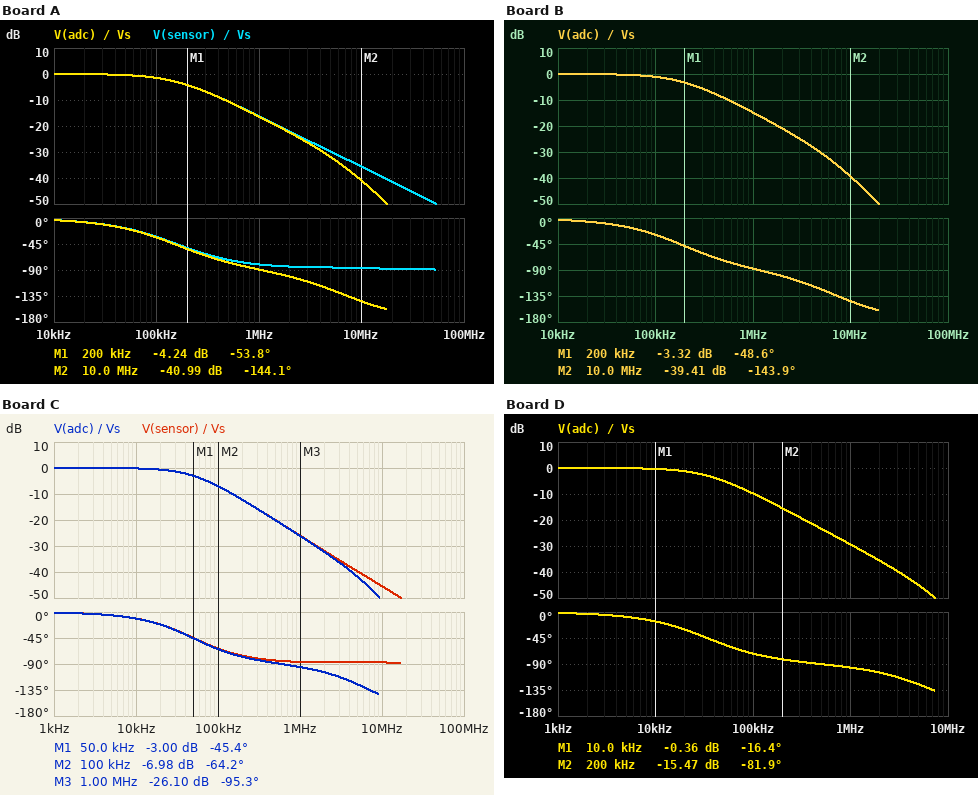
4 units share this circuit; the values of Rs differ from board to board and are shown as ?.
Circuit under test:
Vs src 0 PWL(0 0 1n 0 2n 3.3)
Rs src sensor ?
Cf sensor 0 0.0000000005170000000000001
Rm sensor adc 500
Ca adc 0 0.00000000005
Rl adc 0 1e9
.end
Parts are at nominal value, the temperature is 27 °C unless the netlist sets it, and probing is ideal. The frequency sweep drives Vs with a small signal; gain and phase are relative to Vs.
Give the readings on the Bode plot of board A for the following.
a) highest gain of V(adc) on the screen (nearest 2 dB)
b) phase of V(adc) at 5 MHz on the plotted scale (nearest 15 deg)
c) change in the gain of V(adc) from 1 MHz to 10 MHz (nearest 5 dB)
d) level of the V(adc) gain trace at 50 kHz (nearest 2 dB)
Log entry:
0 dB
-120 deg
-25 dB
0 dB
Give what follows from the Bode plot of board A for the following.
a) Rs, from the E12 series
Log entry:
1.8 kΩ
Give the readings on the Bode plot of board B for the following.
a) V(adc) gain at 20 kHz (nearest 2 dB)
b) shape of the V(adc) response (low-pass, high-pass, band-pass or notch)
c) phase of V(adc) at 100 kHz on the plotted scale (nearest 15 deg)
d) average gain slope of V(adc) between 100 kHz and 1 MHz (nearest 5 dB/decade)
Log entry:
0 dB
low-pass
-30 deg
-15 dB/decade
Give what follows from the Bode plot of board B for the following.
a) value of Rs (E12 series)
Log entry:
1.5 kΩ
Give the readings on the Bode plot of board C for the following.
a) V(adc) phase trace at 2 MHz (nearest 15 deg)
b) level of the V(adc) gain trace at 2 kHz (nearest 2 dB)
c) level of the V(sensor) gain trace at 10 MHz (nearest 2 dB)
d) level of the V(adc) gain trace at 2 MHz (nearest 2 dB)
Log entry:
-105 deg
0 dB
-46 dB
-32 dB
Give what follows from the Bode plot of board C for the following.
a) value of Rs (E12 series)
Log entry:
5.6 kΩ
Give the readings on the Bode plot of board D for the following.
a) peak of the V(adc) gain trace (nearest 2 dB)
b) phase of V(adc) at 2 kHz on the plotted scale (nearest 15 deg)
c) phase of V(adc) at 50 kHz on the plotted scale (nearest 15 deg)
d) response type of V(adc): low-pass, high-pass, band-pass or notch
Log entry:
0 dB
0 deg
-60 deg
low-pass
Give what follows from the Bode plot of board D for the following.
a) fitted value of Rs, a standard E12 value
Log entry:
8.2 kΩ
